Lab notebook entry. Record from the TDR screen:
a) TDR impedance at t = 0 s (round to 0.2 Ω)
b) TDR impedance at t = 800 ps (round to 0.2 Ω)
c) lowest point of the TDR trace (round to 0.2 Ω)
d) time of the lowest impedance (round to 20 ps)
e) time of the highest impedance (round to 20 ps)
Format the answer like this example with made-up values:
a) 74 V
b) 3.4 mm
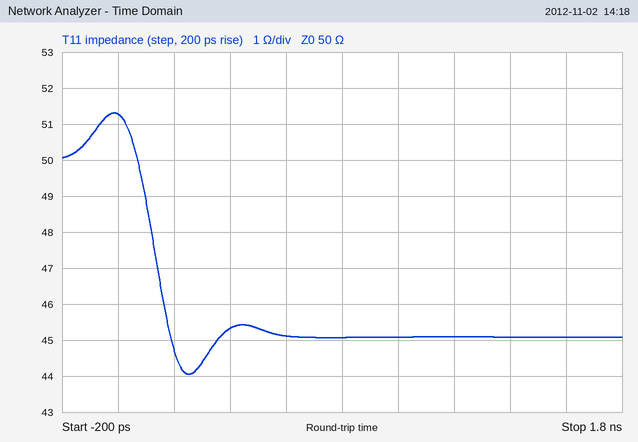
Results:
a) 51.2 Ω
b) 45.0 Ω
c) 44.0 Ω
d) 260 ps
e) -20 ps
